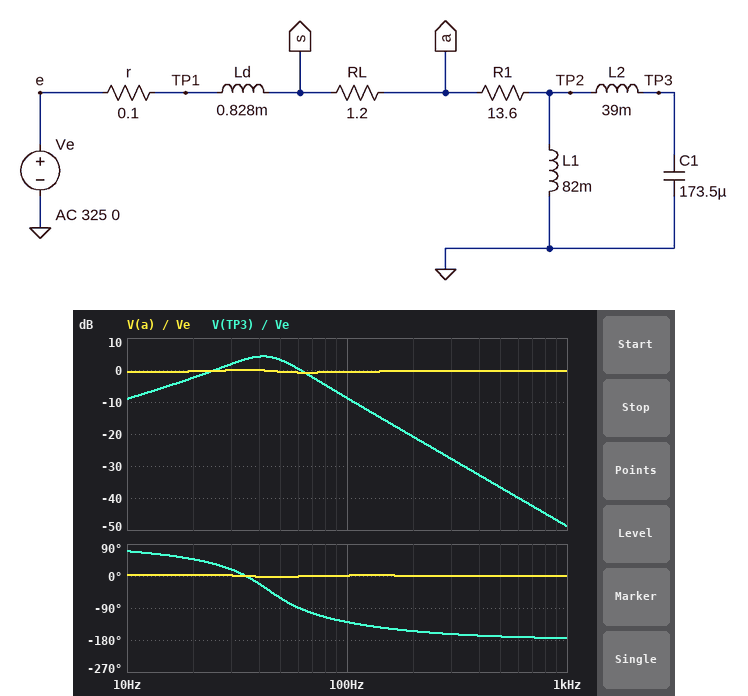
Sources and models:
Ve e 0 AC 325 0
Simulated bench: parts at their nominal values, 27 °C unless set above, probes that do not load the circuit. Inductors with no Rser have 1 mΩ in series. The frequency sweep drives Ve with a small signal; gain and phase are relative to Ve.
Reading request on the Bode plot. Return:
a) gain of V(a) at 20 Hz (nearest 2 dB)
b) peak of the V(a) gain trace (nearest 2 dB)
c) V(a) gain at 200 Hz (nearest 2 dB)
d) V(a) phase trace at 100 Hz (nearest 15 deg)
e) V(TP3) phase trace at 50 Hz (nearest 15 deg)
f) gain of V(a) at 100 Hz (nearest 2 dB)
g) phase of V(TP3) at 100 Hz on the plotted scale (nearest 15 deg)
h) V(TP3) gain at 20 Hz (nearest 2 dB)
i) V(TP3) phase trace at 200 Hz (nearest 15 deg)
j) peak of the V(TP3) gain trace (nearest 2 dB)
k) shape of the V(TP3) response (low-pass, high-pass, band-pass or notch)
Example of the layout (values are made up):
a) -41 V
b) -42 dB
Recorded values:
a) 0 dB
b) 0 dB
c) 0 dB
d) 0 deg
e) -60 deg
f) 0 dB
g) -135 deg
h) -2 dB
i) -150 deg
j) 4 dB
k) band-pass
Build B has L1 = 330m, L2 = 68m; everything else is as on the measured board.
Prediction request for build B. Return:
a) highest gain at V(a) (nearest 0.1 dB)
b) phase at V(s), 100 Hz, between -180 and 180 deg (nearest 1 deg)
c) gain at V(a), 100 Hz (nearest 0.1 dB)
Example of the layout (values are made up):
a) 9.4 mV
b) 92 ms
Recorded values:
a) 0 dB
b) 0 deg
c) -0.3 dB
